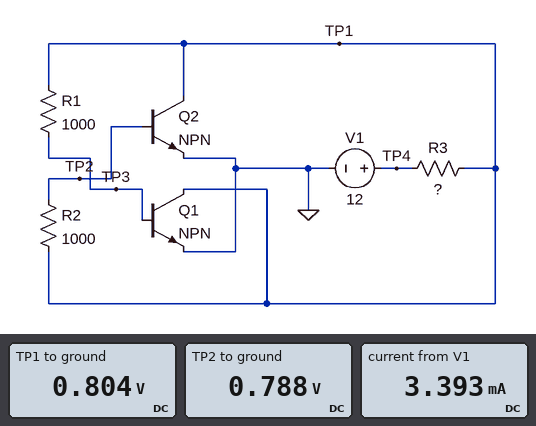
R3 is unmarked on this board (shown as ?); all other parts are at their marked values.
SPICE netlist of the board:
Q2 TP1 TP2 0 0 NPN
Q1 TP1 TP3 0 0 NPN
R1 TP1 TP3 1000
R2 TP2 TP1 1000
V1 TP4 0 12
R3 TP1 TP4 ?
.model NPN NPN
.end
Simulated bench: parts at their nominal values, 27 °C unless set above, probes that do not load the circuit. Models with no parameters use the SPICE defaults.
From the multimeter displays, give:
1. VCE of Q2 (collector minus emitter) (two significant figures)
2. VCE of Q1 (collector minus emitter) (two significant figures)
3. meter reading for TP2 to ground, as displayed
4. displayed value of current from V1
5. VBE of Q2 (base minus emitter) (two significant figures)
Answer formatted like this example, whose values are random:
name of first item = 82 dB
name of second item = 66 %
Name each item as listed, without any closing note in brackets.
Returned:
VCE of Q2 (collector minus emitter) = 800 mV
VCE of Q1 (collector minus emitter) = 800 mV
meter reading for TP2 to ground, as displayed = 0.788 V
displayed value of current from V1 = 3.393 mA
VBE of Q2 (base minus emitter) = 790 mV
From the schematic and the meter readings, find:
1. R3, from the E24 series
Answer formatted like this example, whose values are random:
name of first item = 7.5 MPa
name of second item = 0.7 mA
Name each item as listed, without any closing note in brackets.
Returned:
R3, from the E24 series = 3.3 kΩ
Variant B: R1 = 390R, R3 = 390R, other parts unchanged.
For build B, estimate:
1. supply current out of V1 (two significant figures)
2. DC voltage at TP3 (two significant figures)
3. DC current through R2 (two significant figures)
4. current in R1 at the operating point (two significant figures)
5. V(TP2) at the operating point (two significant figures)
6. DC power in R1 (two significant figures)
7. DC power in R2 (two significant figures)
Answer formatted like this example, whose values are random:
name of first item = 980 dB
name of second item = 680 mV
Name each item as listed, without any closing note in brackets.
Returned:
supply current out of V1 = 28 mA
DC voltage at TP3 = 850 mV
DC current through R2 = 92 µA
current in R1 at the operating point = 190 µA
V(TP2) at the operating point = 830 mV
DC power in R1 = 14 µW
DC power in R2 = 8.5 µW
